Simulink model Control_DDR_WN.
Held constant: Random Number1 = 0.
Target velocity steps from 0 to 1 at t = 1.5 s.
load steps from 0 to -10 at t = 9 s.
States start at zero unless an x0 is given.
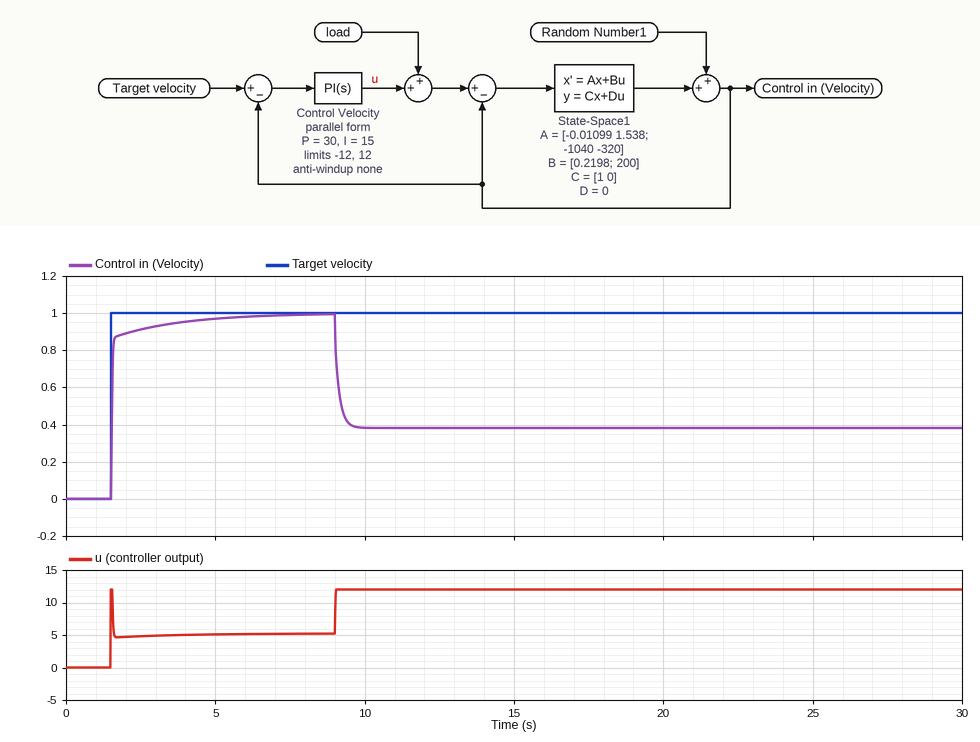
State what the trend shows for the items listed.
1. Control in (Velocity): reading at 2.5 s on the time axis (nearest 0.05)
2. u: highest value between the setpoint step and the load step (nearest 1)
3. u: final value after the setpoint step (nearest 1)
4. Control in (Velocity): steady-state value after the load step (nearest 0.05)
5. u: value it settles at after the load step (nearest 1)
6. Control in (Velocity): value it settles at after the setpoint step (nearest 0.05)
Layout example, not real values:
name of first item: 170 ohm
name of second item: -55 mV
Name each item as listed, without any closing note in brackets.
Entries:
Control in (Velocity): reading at 2.5 s on the time axis: 0.90
u: highest value between the setpoint step and the load step: 12
u: final value after the setpoint step: 5
Control in (Velocity): steady-state value after the load step: 0.40
u: value it settles at after the load step: 12
Control in (Velocity): value it settles at after the setpoint step: 1.00
